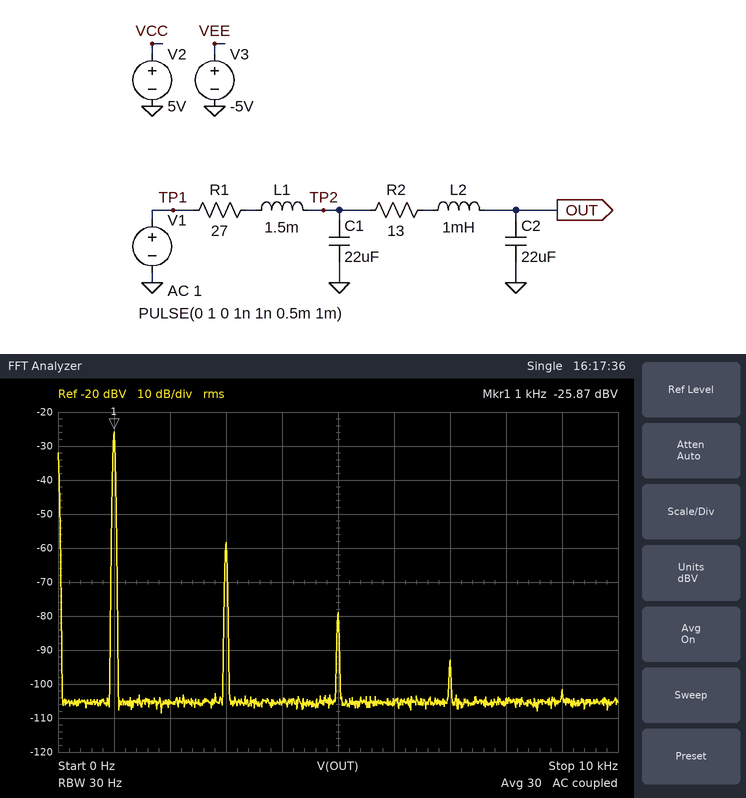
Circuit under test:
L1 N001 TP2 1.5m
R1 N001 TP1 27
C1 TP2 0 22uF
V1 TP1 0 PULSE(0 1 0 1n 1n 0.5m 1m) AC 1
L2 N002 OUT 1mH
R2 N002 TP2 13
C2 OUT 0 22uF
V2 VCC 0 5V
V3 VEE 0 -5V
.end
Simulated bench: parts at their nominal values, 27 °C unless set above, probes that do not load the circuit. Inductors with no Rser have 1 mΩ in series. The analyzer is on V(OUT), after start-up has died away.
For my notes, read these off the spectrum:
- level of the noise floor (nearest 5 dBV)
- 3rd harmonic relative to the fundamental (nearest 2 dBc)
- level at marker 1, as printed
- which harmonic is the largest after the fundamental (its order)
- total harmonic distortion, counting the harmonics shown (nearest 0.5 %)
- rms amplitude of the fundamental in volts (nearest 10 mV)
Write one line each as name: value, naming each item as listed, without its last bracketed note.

level of the noise floor: -105 dBV
3rd harmonic relative to the fundamental: -32 dBc
level at marker 1, as printed: -25.87 dBV
which harmonic is the largest after the fundamental: 3
total harmonic distortion, counting the harmonics shown: 2.5 %
rms amplitude of the fundamental in volts: 50 mV
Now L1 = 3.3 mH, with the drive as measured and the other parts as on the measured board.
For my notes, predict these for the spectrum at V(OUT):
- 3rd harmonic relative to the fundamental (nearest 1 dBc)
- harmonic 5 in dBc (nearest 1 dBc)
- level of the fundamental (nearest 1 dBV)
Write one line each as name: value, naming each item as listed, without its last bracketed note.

3rd harmonic relative to the fundamental: -36 dBc
harmonic 5 in dBc: -58 dBc
level of the fundamental: -27 dBV
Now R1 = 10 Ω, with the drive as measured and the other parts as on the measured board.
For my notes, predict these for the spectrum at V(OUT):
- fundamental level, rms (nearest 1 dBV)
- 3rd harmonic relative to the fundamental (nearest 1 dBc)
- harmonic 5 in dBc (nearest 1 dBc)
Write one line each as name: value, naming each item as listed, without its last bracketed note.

fundamental level, rms: -19 dBV
3rd harmonic relative to the fundamental: -37 dBc
harmonic 5 in dBc: -59 dBc
